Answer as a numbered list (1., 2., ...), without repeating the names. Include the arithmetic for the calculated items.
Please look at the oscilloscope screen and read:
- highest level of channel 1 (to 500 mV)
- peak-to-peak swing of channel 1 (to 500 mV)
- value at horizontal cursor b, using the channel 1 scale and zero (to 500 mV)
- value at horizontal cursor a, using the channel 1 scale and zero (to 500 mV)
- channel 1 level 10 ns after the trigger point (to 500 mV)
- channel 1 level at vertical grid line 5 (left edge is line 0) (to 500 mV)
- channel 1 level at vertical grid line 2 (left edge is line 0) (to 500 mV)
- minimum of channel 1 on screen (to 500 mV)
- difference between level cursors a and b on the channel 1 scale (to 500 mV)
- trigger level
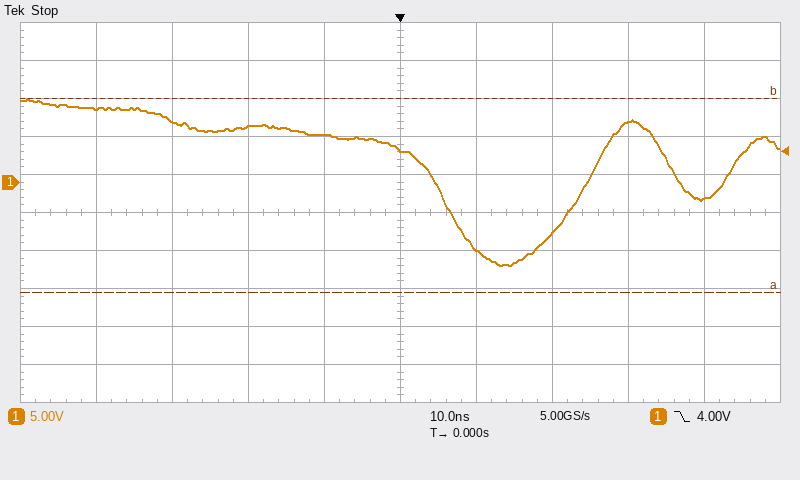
1. 11.0 V
2. 11.0 V − (-11.0 V) = 22.0 V
3. 11.0 V
4. -14.5 V
5. -9.0 V
6. 4.5 V
7. 8.0 V
8. -11.0 V
9. 25.5 V
10. 4.00 V
